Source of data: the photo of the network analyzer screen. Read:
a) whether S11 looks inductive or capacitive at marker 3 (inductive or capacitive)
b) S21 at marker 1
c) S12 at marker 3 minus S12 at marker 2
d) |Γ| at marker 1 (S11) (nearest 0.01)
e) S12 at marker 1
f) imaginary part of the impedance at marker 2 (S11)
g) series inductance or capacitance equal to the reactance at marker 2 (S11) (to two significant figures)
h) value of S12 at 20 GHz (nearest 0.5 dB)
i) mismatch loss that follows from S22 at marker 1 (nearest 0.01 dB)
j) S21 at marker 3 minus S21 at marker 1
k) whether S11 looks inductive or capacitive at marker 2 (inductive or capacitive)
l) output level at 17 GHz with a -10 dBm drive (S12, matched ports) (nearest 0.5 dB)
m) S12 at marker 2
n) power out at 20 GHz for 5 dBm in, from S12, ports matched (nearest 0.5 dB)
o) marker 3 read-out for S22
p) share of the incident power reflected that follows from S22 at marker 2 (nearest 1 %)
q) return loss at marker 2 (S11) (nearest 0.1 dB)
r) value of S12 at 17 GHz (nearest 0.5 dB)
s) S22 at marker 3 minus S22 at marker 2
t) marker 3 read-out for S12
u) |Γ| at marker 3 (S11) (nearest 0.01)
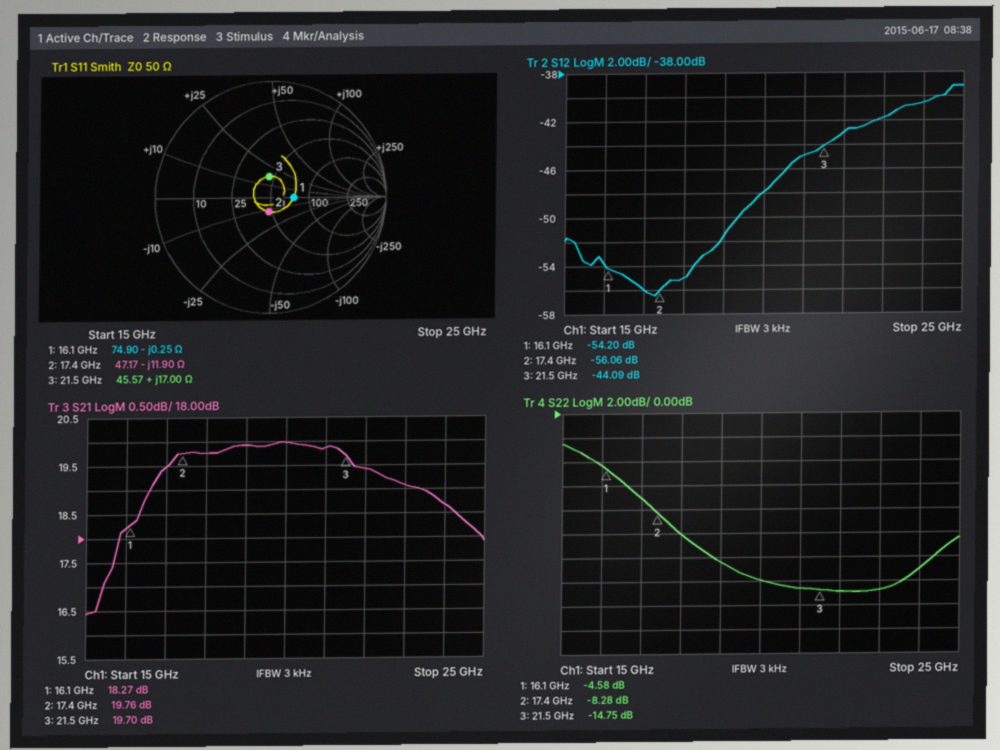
inductive
18.27 dB
11.97 dB
0.20
-54.20 dB
-11.90 Ω
770 fF
-48.0 dB
1.86 dB
1.43 dB
capacitive
-66.0 dBm
-56.06 dB
-43.0 dBm
-14.75 dB
15 %
18.1 dB
-56.0 dB
-6.47 dB
-44.09 dB
0.18
